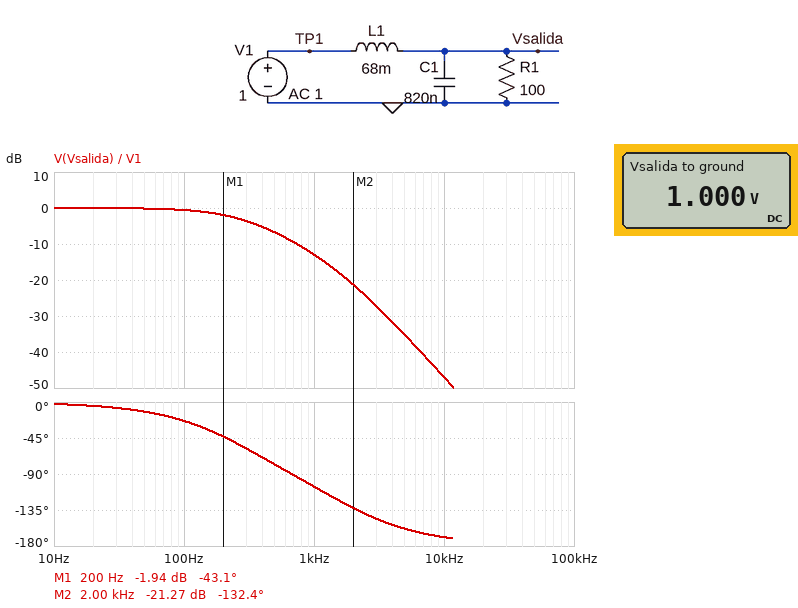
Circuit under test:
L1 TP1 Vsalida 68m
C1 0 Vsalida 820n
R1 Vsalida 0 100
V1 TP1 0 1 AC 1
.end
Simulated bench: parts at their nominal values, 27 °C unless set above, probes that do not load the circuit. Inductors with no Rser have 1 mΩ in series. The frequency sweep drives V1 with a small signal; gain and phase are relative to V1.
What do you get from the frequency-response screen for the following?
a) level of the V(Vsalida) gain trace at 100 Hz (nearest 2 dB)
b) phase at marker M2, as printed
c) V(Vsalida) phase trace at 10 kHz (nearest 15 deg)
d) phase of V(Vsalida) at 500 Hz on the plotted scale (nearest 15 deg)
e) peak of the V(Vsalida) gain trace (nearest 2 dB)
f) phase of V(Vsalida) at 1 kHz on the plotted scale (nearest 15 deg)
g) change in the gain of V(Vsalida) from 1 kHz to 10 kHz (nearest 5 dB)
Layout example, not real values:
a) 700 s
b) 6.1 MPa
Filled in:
a) 0 dB
b) -132.4 deg
c) -165 deg
d) -75 deg
e) 0 dB
f) -105 deg
g) -35 dB
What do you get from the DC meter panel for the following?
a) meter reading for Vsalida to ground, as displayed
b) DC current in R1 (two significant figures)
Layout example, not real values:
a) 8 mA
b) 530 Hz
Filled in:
a) 1.000 V
b) 10 mA
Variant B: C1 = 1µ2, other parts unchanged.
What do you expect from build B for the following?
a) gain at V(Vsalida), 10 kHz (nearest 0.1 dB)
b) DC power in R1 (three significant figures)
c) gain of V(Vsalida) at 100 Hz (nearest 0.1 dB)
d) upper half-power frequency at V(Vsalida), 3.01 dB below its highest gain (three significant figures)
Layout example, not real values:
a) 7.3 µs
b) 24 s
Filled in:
a) -50.2 dB
b) 10.0 mW
c) -0.5 dB
d) 281 Hz
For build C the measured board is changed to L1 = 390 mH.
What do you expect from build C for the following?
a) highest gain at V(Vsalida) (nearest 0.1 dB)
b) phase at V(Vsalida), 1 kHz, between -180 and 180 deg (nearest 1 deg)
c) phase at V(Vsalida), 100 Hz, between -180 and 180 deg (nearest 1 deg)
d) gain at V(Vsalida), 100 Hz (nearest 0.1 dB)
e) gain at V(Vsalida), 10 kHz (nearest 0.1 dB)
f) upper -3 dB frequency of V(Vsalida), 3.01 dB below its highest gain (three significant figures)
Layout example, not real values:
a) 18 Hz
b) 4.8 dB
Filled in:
a) 0 dB
b) -115 deg
c) -70 deg
d) -8.3 dB
e) -62.2 dB
f) 41.7 Hz
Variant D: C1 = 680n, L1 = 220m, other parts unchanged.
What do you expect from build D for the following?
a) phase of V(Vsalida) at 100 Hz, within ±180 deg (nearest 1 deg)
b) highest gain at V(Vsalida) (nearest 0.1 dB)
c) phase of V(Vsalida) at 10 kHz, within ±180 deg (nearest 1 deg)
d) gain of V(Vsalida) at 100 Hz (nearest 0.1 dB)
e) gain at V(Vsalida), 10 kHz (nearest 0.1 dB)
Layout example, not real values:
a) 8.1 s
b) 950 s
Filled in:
a) -56 deg
b) 0 dB
c) -167 deg
d) -4.5 dB
e) -55.6 dB
